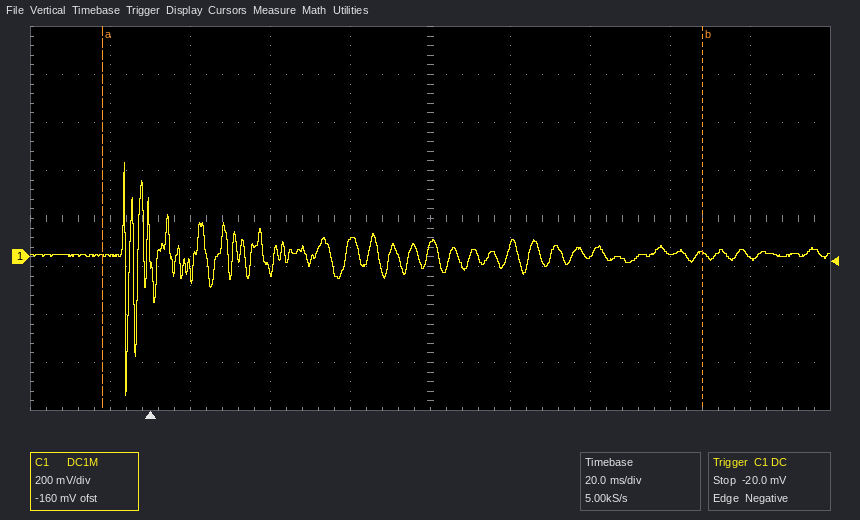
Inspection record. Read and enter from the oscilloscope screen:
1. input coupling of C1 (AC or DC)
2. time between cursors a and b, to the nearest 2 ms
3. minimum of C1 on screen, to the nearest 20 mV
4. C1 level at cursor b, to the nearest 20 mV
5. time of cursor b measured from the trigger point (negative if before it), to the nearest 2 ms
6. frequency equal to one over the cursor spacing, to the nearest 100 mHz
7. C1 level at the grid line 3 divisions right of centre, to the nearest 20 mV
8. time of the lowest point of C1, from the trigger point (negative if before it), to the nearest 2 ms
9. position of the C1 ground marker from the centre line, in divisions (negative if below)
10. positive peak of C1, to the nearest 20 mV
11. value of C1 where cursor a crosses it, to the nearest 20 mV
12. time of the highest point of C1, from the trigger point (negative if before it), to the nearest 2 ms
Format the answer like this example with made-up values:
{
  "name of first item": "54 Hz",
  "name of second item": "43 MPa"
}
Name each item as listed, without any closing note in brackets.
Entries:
{
  "input coupling of C1": "DC",
  "time between cursors a and b, to the nearest 2 ms": "150 ms",
  "minimum of C1 on screen, to the nearest 20 mV": "-580 mV",
  "C1 level at cursor b, to the nearest 20 mV": "20 mV",
  "time of cursor b measured from the trigger point (negative if before it), to the nearest 2 ms": "+138 ms",
  "frequency equal to one over the cursor spacing, to the nearest 100 mHz": "6.7 Hz",
  "C1 level at the grid line 3 divisions right of centre, to the nearest 20 mV": "20 mV",
  "time of the lowest point of C1, from the trigger point (negative if before it), to the nearest 2 ms": "-6 ms",
  "position of the C1 ground marker from the centre line, in divisions": "-0.8 div",
  "positive peak of C1, to the nearest 20 mV": "400 mV",
  "value of C1 where cursor a crosses it, to the nearest 20 mV": "0 mV",
  "time of the highest point of C1, from the trigger point (negative if before it), to the nearest 2 ms": "-6 ms"
}
